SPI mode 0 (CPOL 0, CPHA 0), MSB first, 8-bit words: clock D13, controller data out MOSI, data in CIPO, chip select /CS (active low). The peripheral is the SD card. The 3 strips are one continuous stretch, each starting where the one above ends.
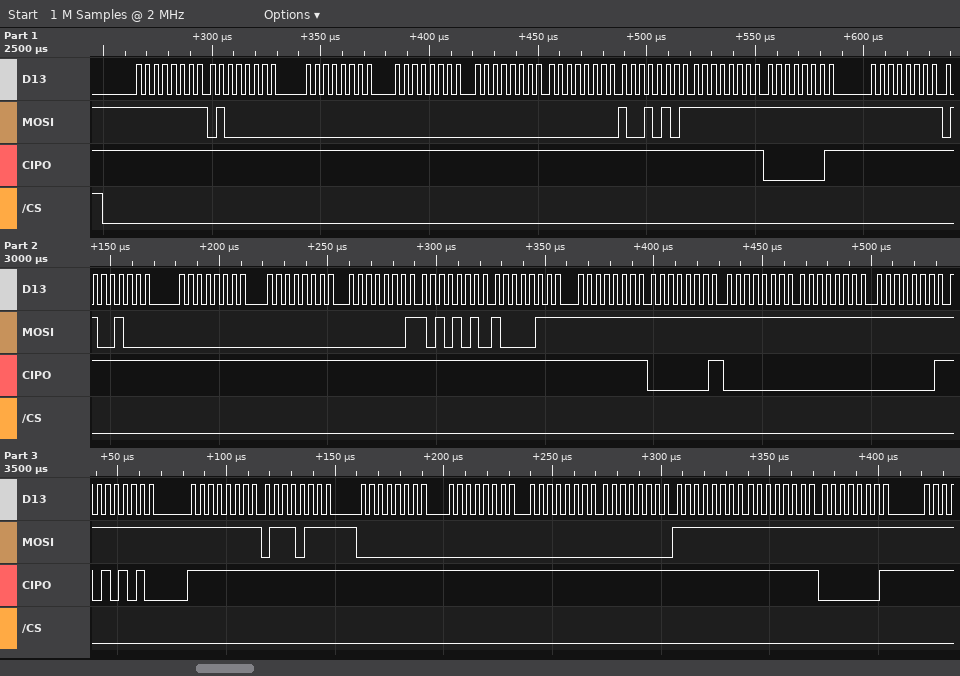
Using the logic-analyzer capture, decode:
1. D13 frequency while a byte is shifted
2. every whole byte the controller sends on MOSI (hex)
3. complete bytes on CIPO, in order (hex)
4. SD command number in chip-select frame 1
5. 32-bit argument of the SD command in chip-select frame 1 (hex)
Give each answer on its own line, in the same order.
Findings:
250 kHz
0xFF 0x40 0x00 0x00 0x00 0x00 0x95 0xFF 0xFF 0xFF 0x48 0x00 0x00 0x01 0xAA 0x87 0xFF 0xFF 0xFF 0xFF 0xFF 0xFF 0xFF 0x77 0x00 0x00 0x00 0x00 0xFF 0xFF 0xFF
0xFF 0xFF 0xFF 0xFF 0xFF 0xFF 0xFF 0xFF 0x01 0xFF 0xFF 0xFF 0xFF 0xFF 0xFF 0xFF 0xFF 0x01 0x00 0x00 0x01 0xAA 0xFF 0xFF 0xFF 0xFF 0xFF 0xFF 0xFF 0xFF 0x01
CMD0
0x00000000
